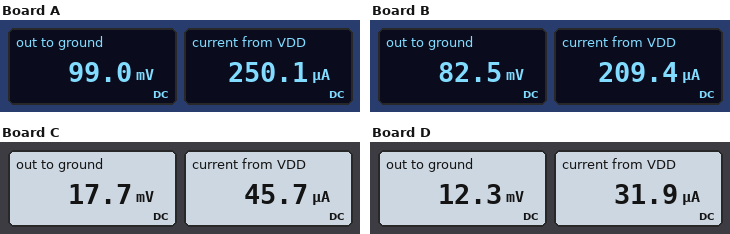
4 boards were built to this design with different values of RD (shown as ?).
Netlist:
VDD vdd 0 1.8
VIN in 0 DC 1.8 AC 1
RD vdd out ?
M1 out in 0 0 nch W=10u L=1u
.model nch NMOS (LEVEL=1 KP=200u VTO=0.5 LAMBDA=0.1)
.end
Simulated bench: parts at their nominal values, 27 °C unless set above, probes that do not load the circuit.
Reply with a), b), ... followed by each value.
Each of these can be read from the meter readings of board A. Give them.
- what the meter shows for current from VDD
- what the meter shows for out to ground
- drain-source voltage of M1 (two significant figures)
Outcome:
a) 250.1 µA
b) 99.0 mV
c) 99 mV
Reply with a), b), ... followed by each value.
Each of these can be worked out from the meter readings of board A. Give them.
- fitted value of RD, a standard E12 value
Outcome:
a) 6.8 kΩ
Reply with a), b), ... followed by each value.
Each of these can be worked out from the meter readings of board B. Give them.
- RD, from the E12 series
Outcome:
a) 8.2 kΩ
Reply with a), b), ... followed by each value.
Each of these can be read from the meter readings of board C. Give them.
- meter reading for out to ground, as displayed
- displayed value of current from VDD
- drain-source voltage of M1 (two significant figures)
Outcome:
a) 17.7 mV
b) 45.7 µA
c) 18 mV
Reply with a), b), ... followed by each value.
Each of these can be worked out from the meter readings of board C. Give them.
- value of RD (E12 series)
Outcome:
a) 39 kΩ
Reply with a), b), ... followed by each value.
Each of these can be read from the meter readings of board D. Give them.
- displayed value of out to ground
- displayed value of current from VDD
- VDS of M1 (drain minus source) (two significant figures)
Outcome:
a) 12.3 mV
b) 31.9 µA
c) 12 mV
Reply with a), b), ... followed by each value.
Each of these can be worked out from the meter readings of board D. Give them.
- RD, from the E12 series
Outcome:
a) 56 kΩ
